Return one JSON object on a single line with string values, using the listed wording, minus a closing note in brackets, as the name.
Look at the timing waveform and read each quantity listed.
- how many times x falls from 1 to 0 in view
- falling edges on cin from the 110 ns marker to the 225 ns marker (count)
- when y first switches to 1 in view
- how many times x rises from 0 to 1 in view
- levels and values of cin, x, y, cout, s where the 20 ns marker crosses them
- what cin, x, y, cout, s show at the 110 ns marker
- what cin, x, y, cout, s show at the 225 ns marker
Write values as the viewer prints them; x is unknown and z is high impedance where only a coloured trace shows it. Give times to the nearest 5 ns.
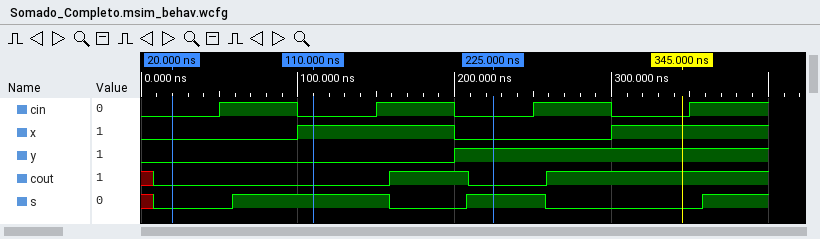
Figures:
{"how many times x falls from 1 to 0 in view": "1", "falling edges on cin from the 110 ns marker to the 225 ns marker": "1", "when y first switches to 1 in view": "200 ns", "how many times x rises from 0 to 1 in view": "2", "levels and values of cin, x, y, cout, s where the 20 ns marker crosses them": "cin=0, x=0, y=0, cout=0, s=0", "what cin, x, y, cout, s show at the 110 ns marker": "cin=0, x=1, y=0, cout=0, s=1", "what cin, x, y, cout, s show at the 225 ns marker": "cin=0, x=0, y=1, cout=0, s=1"}
